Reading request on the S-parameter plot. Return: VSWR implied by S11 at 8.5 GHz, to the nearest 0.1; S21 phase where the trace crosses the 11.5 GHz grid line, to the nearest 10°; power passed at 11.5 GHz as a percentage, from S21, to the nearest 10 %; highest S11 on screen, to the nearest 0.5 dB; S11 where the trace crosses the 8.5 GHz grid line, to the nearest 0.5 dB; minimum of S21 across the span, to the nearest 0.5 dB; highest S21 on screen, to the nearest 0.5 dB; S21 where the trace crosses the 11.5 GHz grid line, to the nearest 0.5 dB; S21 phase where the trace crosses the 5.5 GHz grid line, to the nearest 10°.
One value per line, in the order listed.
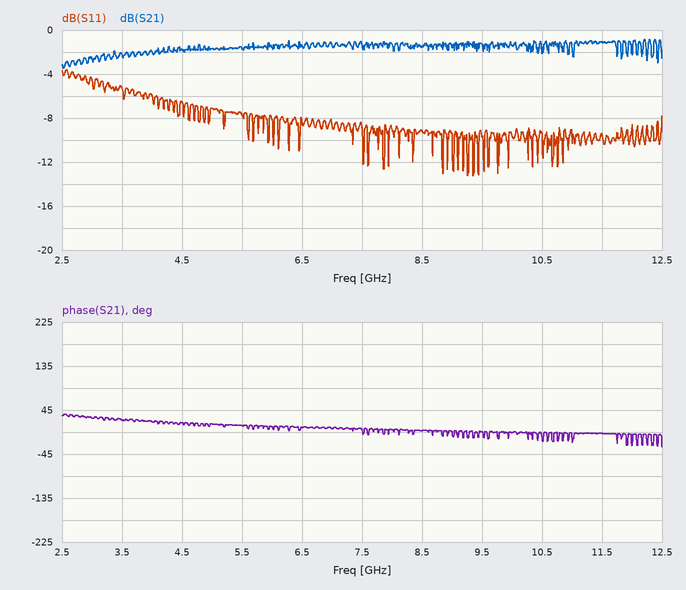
2.1
0°
80 %
-3.5 dB
-9.0 dB
-3.5 dB
-1.0 dB
-1.0 dB
10°
